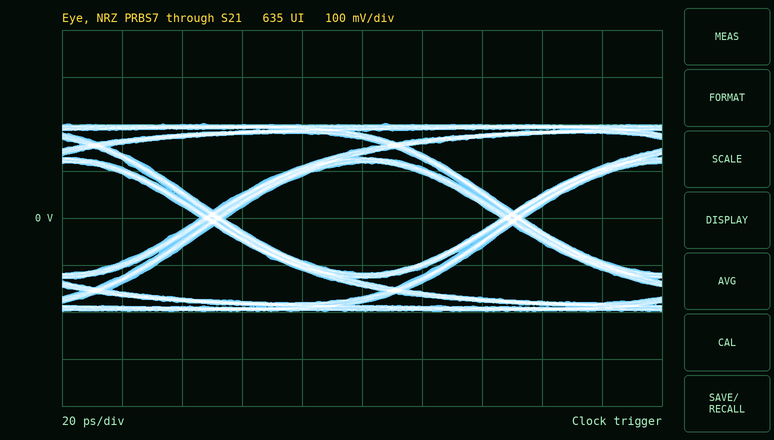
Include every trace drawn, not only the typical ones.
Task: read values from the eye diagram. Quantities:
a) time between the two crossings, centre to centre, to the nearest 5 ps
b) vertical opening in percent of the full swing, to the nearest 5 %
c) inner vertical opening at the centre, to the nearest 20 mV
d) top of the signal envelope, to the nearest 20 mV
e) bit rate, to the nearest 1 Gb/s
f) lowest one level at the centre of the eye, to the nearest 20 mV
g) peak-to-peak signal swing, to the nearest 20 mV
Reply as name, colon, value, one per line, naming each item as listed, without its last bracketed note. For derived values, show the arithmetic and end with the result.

time between the two crossings, centre to centre, to the nearest 5 ps: 100 ps
vertical opening in percent of the full swing, to the nearest 5 %: 240 mV / 400 mV ≈ 60 %
inner vertical opening at the centre, to the nearest 20 mV: 240 mV
top of the signal envelope, to the nearest 20 mV: 200 mV
bit rate, to the nearest 1 Gb/s: 10 Gb/s
lowest one level at the centre of the eye, to the nearest 20 mV: 120 mV
peak-to-peak signal swing, to the nearest 20 mV: 400 mV
